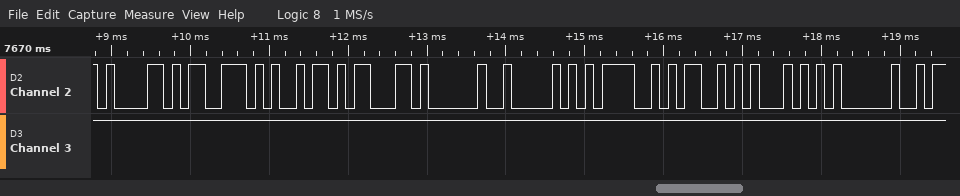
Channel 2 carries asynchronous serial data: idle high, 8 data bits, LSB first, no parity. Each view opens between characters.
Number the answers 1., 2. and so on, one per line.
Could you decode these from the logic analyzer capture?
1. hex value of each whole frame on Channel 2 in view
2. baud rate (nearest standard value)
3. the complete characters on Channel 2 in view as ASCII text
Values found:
1. 61, 73, 69, 63, 20, 50, 4F, 53, 54, 20
2. 9600 baud
3. "asic POST "
